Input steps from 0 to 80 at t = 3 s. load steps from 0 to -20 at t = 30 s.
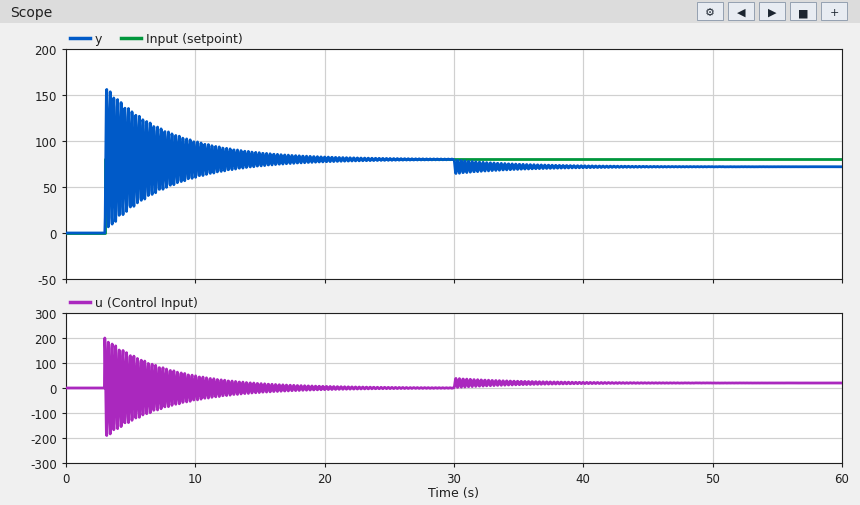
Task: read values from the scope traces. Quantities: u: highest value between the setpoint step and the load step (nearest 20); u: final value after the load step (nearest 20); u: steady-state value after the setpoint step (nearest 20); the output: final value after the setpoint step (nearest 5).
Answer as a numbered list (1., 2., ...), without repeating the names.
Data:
1. 200
2. 20
3. 0
4. 80
